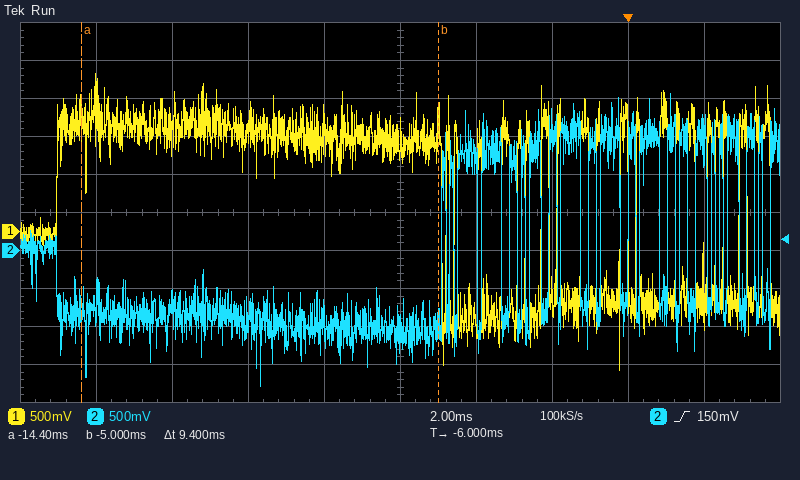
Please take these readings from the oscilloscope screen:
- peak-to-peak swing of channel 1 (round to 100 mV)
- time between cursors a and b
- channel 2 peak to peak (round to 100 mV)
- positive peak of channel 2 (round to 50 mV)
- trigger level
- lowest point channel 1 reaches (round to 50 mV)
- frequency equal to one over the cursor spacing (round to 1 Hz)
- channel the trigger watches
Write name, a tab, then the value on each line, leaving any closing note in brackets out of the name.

peak-to-peak swing of channel 1	3.90 V
time between cursors a and b	9.4 ms
channel 2 peak to peak	3.80 V
positive peak of channel 2	2.05 V
trigger level	150 mV
lowest point channel 1 reaches	-1.80 V
frequency equal to one over the cursor spacing	106 Hz
channel the trigger watches	channel 2
